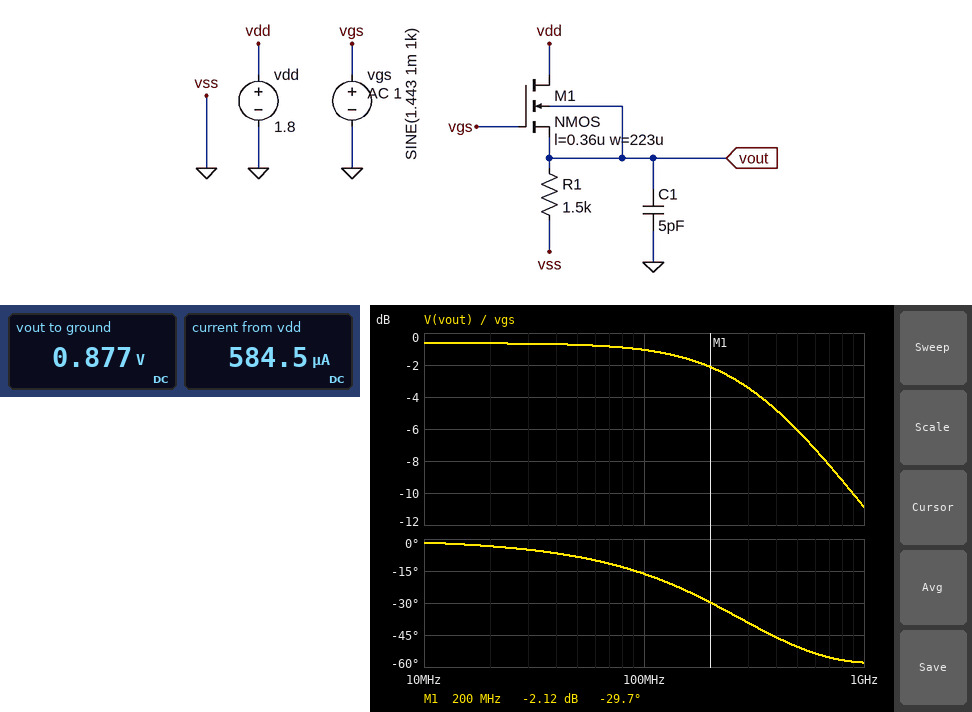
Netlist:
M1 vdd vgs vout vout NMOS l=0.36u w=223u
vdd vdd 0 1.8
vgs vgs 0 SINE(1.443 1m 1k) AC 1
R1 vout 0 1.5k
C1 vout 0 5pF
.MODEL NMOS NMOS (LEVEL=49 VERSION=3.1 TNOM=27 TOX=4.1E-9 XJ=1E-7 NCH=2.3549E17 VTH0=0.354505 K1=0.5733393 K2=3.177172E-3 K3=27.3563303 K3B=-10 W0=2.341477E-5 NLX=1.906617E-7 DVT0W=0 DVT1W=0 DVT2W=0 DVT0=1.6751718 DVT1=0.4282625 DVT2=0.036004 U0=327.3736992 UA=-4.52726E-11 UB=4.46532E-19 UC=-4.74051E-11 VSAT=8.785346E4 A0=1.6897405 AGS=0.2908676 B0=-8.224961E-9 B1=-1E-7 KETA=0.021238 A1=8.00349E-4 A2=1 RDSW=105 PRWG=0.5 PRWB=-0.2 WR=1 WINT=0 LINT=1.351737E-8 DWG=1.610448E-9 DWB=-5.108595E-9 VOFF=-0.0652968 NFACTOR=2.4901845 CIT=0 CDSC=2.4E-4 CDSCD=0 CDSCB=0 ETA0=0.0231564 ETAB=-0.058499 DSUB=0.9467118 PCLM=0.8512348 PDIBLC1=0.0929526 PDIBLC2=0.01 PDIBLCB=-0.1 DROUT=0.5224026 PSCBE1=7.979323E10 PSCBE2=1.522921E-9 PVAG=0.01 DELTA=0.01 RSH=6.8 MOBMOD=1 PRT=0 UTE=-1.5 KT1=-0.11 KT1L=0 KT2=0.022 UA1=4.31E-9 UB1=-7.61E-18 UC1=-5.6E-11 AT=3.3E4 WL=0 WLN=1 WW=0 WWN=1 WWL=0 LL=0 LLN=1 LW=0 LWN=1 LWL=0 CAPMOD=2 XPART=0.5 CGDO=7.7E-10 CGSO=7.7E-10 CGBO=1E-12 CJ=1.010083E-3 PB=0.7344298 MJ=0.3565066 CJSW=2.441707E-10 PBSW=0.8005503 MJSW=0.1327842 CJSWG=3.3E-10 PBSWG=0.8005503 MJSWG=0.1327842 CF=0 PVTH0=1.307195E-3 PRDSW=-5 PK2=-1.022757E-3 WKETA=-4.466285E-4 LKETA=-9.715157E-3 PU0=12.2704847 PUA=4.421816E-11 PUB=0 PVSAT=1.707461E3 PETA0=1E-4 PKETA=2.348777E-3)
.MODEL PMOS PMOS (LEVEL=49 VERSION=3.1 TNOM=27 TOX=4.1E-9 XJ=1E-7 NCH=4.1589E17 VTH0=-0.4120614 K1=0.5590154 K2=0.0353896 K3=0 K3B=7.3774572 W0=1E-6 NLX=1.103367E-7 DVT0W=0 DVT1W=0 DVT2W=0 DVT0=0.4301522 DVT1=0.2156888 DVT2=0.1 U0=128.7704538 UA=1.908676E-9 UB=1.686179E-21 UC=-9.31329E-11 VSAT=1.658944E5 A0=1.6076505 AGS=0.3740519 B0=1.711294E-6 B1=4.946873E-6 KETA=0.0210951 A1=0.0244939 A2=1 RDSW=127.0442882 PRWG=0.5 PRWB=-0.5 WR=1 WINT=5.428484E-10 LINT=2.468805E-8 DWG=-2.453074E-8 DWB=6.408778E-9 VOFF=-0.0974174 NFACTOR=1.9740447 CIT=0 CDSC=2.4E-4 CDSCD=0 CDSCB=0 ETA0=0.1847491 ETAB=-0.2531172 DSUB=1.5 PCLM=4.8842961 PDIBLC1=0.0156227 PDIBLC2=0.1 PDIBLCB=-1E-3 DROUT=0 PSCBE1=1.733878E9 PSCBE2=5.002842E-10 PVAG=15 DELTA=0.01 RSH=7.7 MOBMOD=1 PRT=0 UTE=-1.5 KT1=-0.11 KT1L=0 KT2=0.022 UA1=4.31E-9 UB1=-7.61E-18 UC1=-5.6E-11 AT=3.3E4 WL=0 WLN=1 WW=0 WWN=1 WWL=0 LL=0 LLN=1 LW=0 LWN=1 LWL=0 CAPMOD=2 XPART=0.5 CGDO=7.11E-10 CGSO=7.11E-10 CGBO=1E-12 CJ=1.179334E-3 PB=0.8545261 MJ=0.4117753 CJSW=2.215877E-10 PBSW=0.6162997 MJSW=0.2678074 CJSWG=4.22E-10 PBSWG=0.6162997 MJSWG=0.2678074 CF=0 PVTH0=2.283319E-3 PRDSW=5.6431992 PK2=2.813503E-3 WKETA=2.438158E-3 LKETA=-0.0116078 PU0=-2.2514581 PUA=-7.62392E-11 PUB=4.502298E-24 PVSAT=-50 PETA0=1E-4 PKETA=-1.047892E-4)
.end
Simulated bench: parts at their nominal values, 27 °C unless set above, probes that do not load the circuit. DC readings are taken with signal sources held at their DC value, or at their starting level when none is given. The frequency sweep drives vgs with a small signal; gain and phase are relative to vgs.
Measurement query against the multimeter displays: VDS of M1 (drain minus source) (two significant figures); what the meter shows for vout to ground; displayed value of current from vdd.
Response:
920 mV
0.877 V
584.5 µA
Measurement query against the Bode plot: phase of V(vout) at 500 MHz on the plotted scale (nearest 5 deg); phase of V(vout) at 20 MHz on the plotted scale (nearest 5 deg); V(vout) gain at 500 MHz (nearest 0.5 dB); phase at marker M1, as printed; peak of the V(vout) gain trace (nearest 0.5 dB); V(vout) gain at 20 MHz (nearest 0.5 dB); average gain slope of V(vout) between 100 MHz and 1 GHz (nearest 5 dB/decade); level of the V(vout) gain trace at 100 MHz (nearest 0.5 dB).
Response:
-50 deg
-5 deg
-6.0 dB
-29.7 deg
-0.5 dB
-0.5 dB
-10 dB/decade
-1.0 dB
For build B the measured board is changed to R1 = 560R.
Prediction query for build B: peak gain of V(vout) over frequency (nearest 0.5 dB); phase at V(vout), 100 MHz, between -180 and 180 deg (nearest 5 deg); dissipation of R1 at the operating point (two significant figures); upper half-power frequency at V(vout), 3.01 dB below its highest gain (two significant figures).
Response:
-1.0 dB
-10 deg
1.2 mW
580 MHz
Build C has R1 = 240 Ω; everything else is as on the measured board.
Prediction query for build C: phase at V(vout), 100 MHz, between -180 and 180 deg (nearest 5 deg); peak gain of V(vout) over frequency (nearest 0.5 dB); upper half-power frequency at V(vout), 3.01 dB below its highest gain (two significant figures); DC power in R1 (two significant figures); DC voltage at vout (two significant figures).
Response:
-5 deg
-1.5 dB
860 MHz
2.3 mW
740 mV
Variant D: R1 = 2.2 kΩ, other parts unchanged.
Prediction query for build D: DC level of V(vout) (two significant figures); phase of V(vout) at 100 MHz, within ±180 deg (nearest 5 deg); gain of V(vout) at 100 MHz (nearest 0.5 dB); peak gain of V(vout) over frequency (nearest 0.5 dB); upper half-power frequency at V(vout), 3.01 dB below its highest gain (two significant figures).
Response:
900 mV
-20 deg
-1.5 dB
-0.5 dB
240 MHz
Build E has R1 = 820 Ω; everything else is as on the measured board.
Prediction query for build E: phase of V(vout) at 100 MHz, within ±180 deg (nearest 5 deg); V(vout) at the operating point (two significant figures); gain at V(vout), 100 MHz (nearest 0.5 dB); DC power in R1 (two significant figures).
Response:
-10 deg
840 mV
-1.0 dB
860 µW
